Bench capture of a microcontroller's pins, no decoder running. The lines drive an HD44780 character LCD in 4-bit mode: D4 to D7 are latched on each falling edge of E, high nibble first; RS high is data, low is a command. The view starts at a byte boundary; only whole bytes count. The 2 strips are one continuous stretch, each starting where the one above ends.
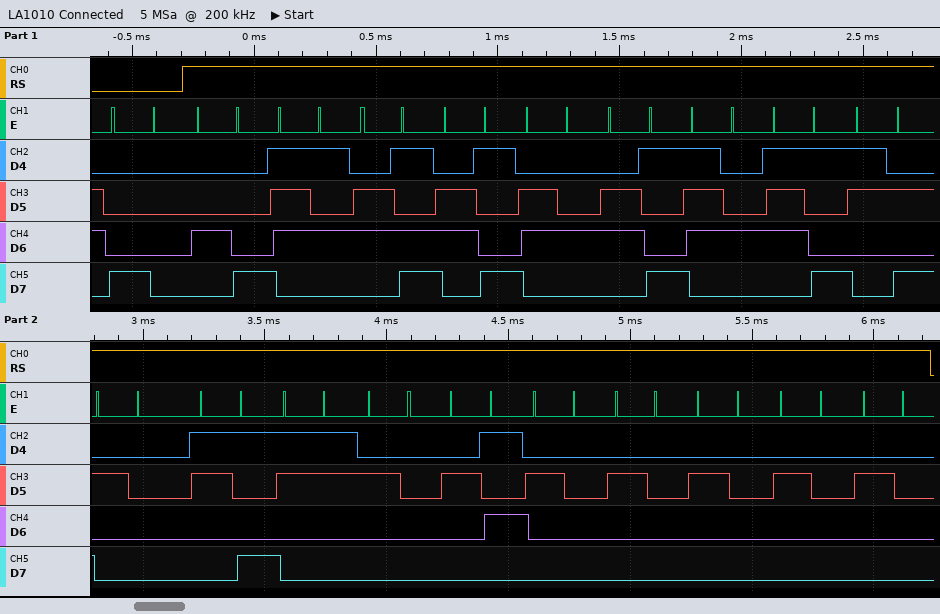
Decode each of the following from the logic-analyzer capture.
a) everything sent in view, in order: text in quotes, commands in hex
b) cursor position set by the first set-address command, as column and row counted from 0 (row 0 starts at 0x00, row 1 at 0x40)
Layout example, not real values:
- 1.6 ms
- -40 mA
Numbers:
- 0x80 "Humidity: 93 %     "
- column 0, row 0
